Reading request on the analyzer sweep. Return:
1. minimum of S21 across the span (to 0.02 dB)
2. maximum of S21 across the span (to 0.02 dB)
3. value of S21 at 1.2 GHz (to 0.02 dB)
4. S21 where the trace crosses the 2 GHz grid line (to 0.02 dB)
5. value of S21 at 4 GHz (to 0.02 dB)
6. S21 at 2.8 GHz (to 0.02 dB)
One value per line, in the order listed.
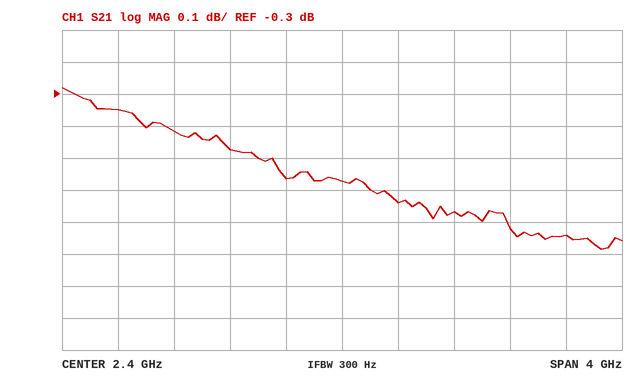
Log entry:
-0.78 dB
-0.28 dB
-0.42 dB
-0.56 dB
-0.74 dB
-0.64 dB
